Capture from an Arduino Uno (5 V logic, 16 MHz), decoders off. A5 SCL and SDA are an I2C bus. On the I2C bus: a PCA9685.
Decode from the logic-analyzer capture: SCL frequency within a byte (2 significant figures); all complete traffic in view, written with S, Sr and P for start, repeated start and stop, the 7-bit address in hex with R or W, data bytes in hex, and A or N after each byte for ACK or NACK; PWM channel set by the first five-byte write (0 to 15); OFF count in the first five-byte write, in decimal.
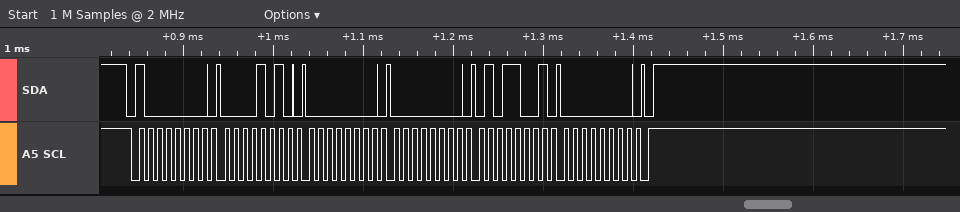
100 kHz
S 40W A 0A A 00 A 00 A 59 A 00 A P
1
89
